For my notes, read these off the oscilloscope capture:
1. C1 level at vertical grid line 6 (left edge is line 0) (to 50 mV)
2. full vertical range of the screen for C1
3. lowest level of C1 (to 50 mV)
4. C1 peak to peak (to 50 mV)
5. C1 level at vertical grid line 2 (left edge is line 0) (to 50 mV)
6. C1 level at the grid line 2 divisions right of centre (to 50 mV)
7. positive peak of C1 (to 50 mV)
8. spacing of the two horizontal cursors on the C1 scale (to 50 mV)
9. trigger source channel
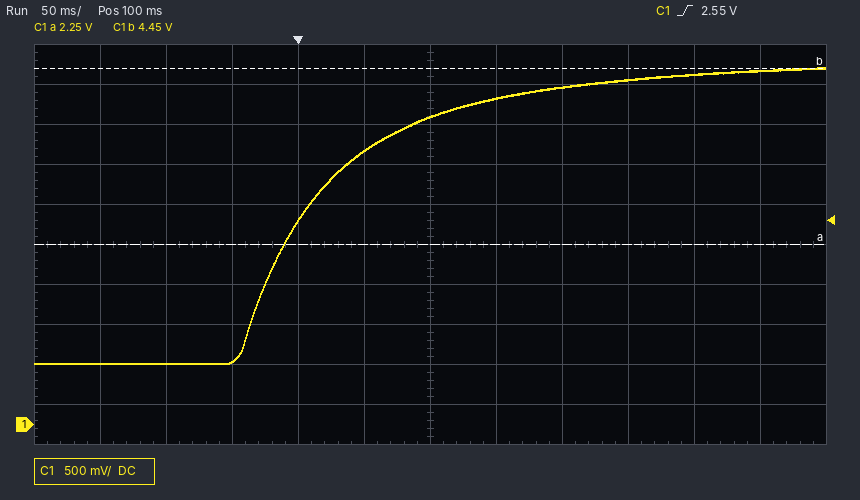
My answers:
3.85 V
5 V
750 mV
3.70 V
750 mV
4.20 V
4.45 V
2.20 V
C1
